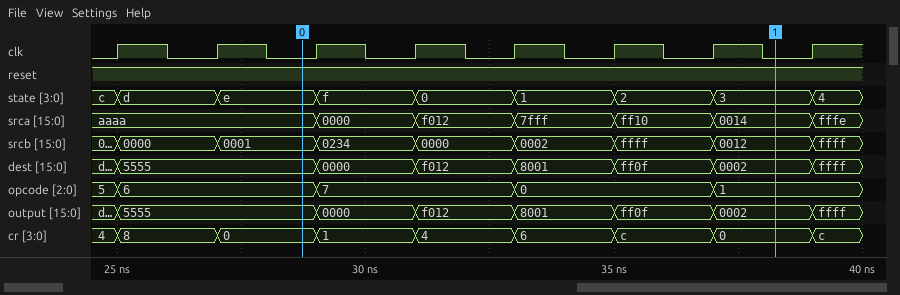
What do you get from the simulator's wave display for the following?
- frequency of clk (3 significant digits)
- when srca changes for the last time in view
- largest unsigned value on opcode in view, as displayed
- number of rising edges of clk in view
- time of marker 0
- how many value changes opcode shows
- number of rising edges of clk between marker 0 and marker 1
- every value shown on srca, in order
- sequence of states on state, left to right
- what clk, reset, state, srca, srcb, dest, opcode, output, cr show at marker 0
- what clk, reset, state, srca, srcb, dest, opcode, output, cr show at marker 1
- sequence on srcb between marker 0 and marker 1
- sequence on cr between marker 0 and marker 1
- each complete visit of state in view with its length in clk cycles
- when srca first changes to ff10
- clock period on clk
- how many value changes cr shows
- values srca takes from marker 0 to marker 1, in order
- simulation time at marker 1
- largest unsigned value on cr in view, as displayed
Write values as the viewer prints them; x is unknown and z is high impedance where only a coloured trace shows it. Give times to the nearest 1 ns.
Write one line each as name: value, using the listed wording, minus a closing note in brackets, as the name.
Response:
frequency of clk: 500 MHz
when srca changes for the last time in view: 39 ns
largest unsigned value on opcode in view, as displayed: 7
number of rising edges of clk in view: 8
time of marker 0: 29 ns
how many value changes opcode shows: 4
number of rising edges of clk between marker 0 and marker 1: 5
every value shown on srca, in order: aaaa, 0000, f012, 7fff, ff10, 0014, fffe
sequence of states on state, left to right: c, d, e, f, 0, 1, 2, 3, 4
what clk, reset, state, srca, srcb, dest, opcode, output, cr show at marker 0: clk=0, reset=1, state=e, srca=aaaa, srcb=0001, dest=5555, opcode=6, output=5555, cr=0
what clk, reset, state, srca, srcb, dest, opcode, output, cr show at marker 1: clk=0, reset=1, state=3, srca=0014, srcb=0012, dest=0002, opcode=1, output=0002, cr=0
sequence on srcb between marker 0 and marker 1: 0001, 0234, 0000, 0002, ffff, 0012
sequence on cr between marker 0 and marker 1: 0, 1, 4, 6, c, 0
each complete visit of state in view with its length in clk cycles: d: 1, e: 1, f: 1, 0: 1, 1: 1, 2: 1, 3: 1
when srca first changes to ff10: 35 ns
clock period on clk: 2 ns
how many value changes cr shows: 8
values srca takes from marker 0 to marker 1, in order: aaaa, 0000, f012, 7fff, ff10, 0014
simulation time at marker 1: 38 ns
largest unsigned value on cr in view, as displayed: c
